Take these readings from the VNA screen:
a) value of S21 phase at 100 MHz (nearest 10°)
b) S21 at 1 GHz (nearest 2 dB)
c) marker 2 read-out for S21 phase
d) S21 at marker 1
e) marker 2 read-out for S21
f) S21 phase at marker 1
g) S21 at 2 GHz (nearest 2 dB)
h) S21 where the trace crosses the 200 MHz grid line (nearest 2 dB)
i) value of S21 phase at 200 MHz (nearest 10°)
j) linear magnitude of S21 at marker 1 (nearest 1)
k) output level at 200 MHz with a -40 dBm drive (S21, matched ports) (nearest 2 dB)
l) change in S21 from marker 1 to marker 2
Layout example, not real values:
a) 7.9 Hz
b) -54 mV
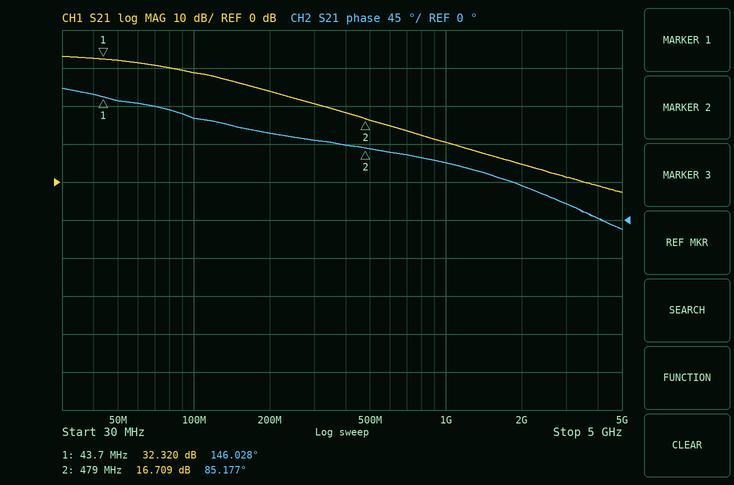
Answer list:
a) 120°
b) 10 dB
c) 85.177°
d) 32.320 dB
e) 16.709 dB
f) 146.028°
g) 4 dB
h) 24 dB
i) 100°
j) 41
k) -16 dBm
l) -15.611 dB
